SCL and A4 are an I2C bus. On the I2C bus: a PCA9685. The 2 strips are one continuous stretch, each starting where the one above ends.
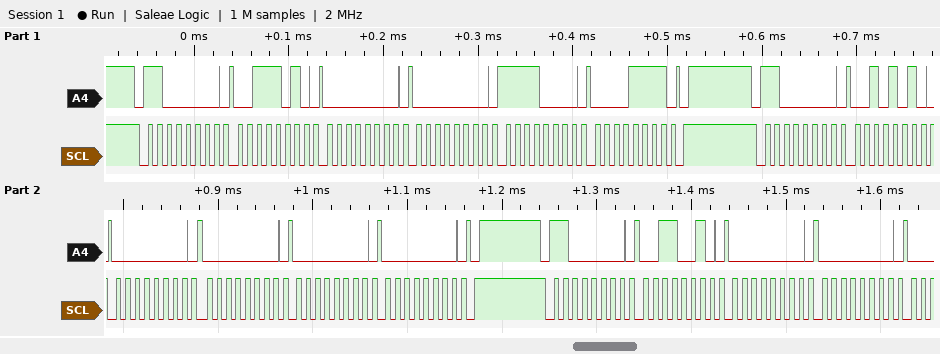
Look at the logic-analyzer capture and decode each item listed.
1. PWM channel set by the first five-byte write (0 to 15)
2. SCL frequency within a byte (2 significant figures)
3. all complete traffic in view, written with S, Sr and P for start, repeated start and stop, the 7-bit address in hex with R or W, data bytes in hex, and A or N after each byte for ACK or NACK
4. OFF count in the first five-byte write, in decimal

13
100 kHz
S 60W A 3A A 00 A 00 A F0 A 0F A P S 60W A 2A A 00 A 00 A 00 A 00 A P S 60W A 32 A 00 A 00 A
4080
